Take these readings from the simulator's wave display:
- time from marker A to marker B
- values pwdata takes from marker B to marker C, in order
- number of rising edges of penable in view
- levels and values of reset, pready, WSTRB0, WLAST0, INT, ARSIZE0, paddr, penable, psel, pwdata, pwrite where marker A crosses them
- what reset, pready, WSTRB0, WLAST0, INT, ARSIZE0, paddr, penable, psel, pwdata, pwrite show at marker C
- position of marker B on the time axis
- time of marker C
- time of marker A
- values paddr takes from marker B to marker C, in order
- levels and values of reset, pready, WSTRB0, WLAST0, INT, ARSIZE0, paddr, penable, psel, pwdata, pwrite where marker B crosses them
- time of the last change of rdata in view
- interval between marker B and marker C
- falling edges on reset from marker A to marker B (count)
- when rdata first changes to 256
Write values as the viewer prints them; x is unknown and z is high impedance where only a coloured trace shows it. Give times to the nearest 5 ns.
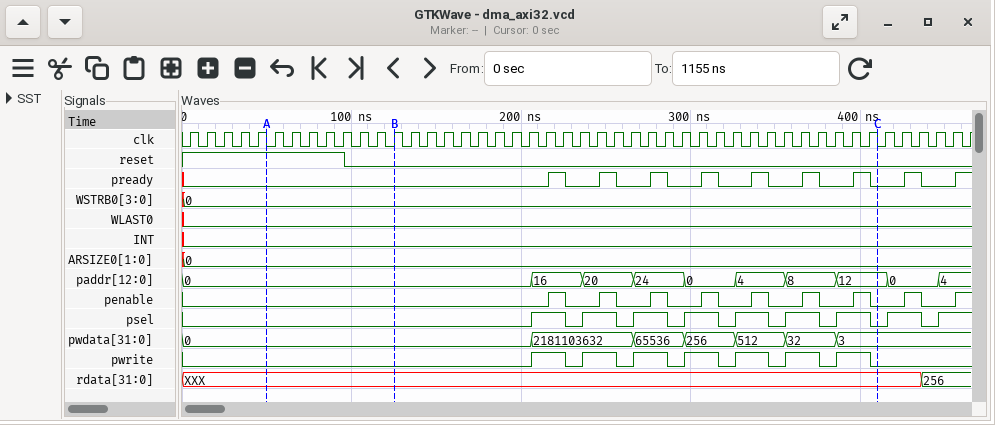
75 ns
0, 2181103632, 65536, 256, 512, 32, 3
9
reset=1, pready=0, WSTRB0=0, WLAST0=0, INT=0, ARSIZE0=0, paddr=0, penable=0, psel=0, pwdata=0, pwrite=0
reset=0, pready=0, WSTRB0=0, WLAST0=0, INT=0, ARSIZE0=0, paddr=12, penable=0, psel=0, pwdata=3, pwrite=0
125 ns
410 ns
50 ns
0, 16, 20, 24, 0, 4, 8, 12
reset=0, pready=0, WSTRB0=0, WLAST0=0, INT=0, ARSIZE0=0, paddr=0, penable=0, psel=0, pwdata=0, pwrite=0
435 ns
285 ns
1
435 ns
